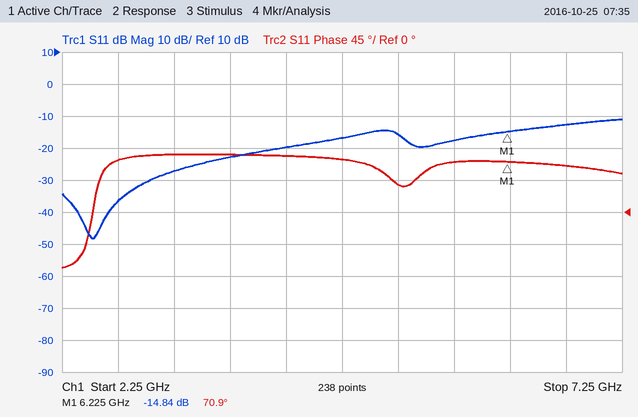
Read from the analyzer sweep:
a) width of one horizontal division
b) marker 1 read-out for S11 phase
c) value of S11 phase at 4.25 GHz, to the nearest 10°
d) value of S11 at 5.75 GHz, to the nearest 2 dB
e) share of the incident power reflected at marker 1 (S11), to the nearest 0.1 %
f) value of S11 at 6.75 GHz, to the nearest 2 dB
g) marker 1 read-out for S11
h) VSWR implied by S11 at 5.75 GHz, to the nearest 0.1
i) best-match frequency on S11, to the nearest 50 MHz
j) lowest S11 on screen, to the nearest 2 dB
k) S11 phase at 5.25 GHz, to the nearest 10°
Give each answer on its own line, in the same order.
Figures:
500 MHz
70.9°
80°
-18 dB
3.3 %
-12 dB
-14.84 dB
1.3
2.50 GHz
-48 dB
40°
